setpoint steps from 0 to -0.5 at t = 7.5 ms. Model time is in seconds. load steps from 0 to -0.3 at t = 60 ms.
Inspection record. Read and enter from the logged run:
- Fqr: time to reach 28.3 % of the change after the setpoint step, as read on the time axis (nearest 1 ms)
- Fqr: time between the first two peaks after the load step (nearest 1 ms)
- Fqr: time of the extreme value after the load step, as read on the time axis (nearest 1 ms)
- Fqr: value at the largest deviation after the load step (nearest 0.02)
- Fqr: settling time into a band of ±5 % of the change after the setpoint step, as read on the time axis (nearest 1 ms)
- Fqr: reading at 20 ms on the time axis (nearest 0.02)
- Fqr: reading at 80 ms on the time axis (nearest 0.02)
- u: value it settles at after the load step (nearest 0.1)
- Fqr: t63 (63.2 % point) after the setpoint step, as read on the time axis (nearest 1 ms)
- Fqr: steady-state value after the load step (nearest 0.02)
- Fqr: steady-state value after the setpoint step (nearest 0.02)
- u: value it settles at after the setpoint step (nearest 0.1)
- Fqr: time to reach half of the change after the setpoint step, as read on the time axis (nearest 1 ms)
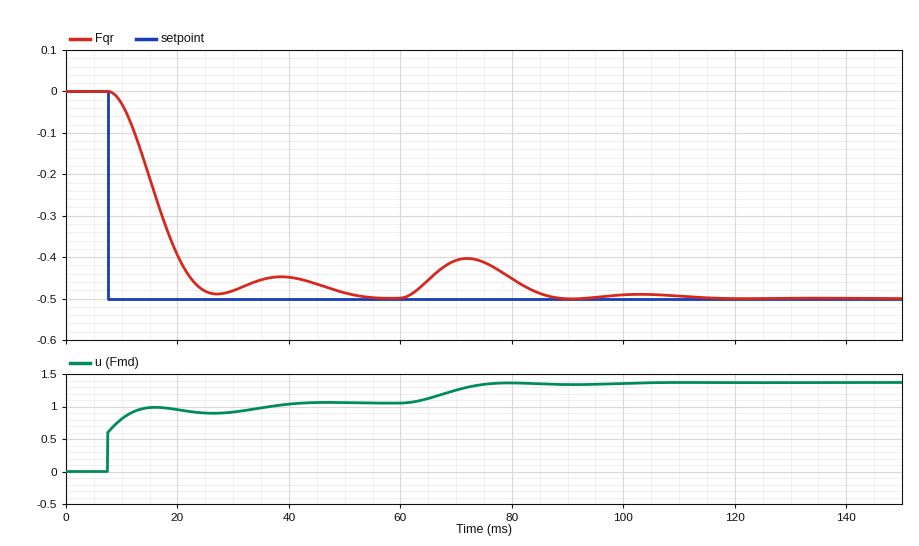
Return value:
13 ms
31 ms
72 ms
-0.40
47 ms
-0.40
-0.46
1.4
18 ms
-0.50
-0.50
1.1
16 ms
